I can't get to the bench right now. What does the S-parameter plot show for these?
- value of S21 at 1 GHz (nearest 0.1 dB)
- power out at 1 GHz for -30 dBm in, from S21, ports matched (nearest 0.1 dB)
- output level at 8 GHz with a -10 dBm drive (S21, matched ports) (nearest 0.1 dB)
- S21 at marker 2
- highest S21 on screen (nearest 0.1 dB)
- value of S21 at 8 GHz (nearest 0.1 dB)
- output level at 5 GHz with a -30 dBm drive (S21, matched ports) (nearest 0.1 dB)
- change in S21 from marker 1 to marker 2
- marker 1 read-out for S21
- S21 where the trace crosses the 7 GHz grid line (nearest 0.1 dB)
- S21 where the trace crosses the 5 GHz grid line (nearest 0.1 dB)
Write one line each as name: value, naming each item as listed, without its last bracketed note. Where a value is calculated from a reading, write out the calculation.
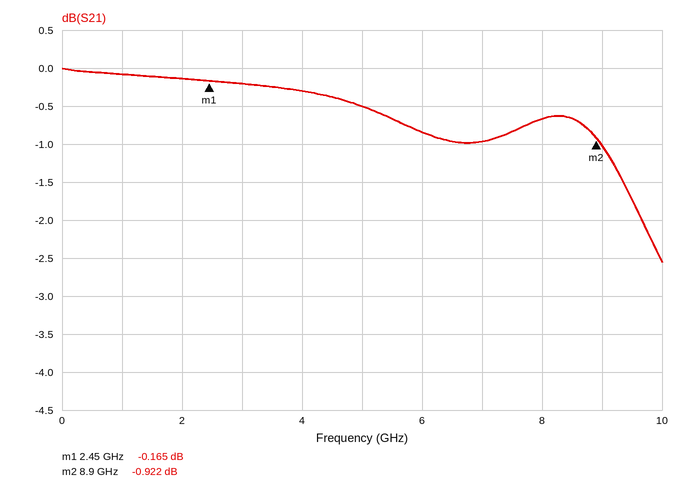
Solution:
value of S21 at 1 GHz: -0.1 dB
power out at 1 GHz for -30 dBm in, from S21, ports matched: -30 dBm + (-0.1 dB) = -30.1 dBm
output level at 8 GHz with a -10 dBm drive (S21, matched ports): -10 dBm + (-0.7 dB) = -10.7 dBm
S21 at marker 2: -0.922 dB
highest S21 on screen: 0.0 dB
value of S21 at 8 GHz: -0.7 dB
output level at 5 GHz with a -30 dBm drive (S21, matched ports): -30 dBm + (-0.5 dB) = -30.5 dBm
change in S21 from marker 1 to marker 2: -0.922 − (-0.165) = -0.757 dB
marker 1 read-out for S21: -0.165 dB
S21 where the trace crosses the 7 GHz grid line: -1.0 dB
S21 where the trace crosses the 5 GHz grid line: -0.5 dB
